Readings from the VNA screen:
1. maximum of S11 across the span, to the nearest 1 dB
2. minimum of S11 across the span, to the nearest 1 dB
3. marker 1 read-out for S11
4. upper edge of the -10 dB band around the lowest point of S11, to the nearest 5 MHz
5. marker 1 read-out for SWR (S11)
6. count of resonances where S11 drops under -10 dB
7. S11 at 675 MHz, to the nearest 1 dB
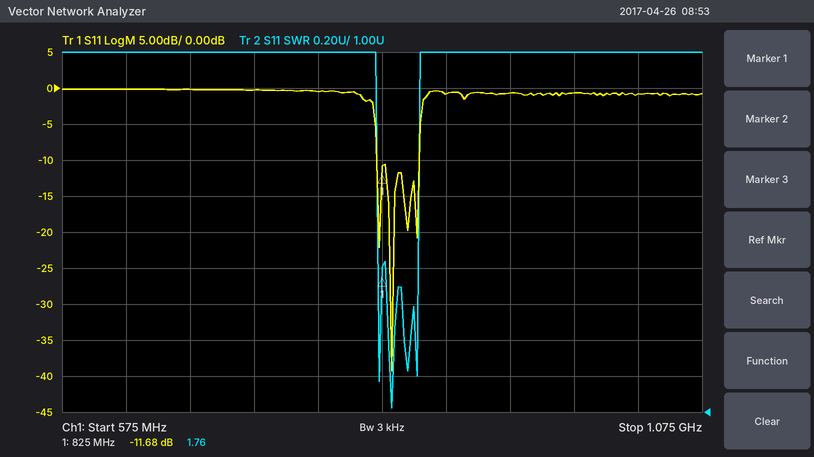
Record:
0 dB
-39 dB
-11.68 dB
855 MHz
1.76
4
0 dB
